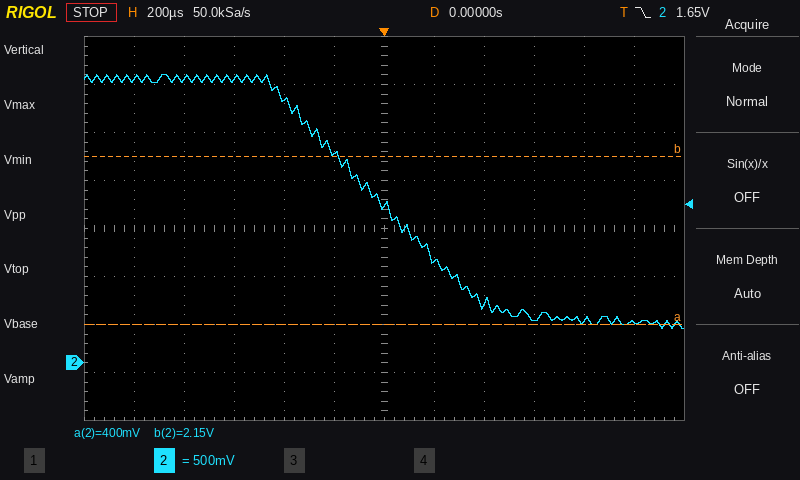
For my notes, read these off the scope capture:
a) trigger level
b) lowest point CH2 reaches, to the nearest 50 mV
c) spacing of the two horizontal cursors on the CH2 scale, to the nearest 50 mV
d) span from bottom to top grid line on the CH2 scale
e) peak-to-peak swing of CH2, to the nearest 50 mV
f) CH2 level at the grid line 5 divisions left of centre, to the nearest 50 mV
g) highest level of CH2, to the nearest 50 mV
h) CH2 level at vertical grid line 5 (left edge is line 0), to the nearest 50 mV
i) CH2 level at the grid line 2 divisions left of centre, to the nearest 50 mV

1.65 V
350 mV
1.75 V
4 V
2.65 V
2.95 V
3.00 V
2.20 V
2.75 V
